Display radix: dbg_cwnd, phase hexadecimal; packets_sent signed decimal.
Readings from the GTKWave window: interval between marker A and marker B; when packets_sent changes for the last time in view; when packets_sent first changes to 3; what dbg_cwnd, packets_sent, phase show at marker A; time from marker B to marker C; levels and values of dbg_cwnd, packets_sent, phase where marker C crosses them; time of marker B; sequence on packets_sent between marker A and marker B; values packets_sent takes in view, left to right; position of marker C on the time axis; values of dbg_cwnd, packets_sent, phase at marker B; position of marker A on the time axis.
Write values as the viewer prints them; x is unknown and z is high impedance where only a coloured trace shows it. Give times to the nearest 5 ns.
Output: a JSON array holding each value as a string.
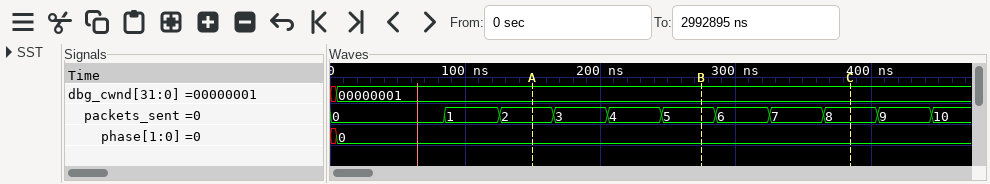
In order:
["125 ns", "445 ns", "165 ns", "dbg_cwnd=00000001, packets_sent=2, phase=0", "110 ns", "dbg_cwnd=00000001, packets_sent=8, phase=0", "275 ns", "2, 3, 4, 5", "0, 1, 2, 3, 4, 5, 6, 7, 8, 9, 10", "385 ns", "dbg_cwnd=00000001, packets_sent=5, phase=0", "150 ns"]
